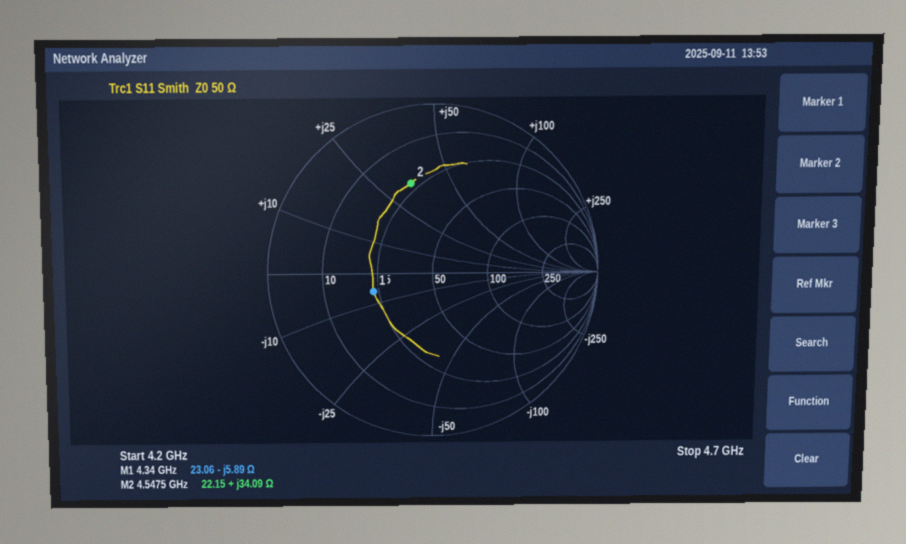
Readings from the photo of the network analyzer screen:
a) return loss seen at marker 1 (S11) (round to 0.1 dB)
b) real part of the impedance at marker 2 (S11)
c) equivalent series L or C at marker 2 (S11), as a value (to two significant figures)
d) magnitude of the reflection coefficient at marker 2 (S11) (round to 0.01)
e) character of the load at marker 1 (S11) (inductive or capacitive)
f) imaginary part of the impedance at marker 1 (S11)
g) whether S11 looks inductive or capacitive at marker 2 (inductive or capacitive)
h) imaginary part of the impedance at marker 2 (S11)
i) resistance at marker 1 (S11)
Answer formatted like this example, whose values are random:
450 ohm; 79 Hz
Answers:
8.5 dB; 22.15 Ω; 1.2 nH; 0.55; capacitive; -5.89 Ω; inductive; +34.09 Ω; 23.06 Ω
